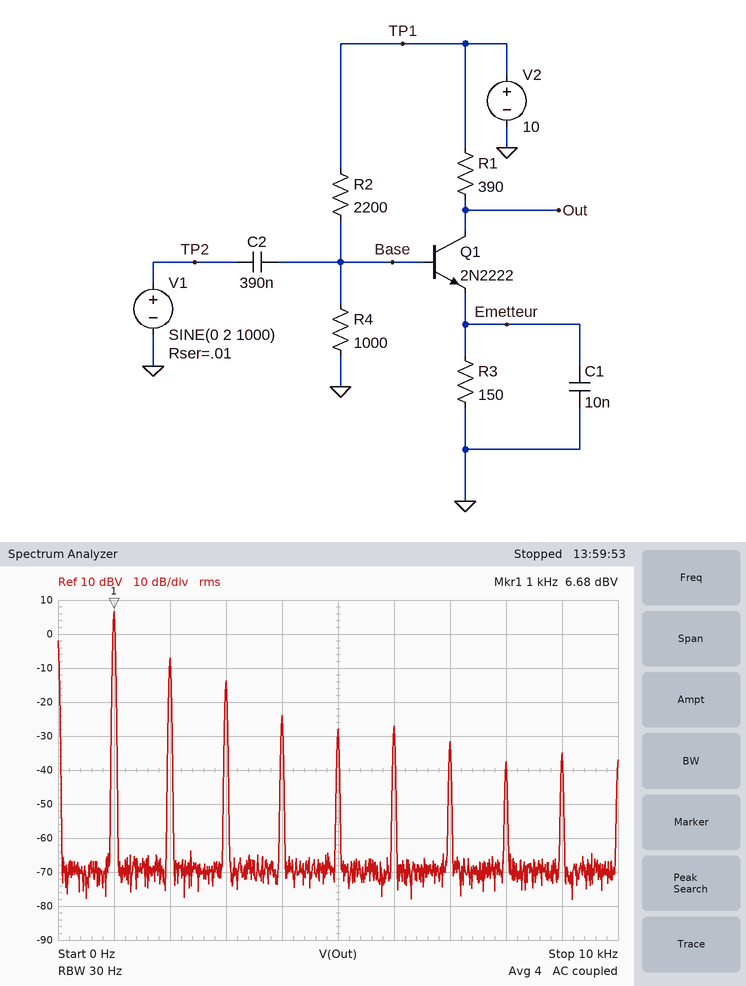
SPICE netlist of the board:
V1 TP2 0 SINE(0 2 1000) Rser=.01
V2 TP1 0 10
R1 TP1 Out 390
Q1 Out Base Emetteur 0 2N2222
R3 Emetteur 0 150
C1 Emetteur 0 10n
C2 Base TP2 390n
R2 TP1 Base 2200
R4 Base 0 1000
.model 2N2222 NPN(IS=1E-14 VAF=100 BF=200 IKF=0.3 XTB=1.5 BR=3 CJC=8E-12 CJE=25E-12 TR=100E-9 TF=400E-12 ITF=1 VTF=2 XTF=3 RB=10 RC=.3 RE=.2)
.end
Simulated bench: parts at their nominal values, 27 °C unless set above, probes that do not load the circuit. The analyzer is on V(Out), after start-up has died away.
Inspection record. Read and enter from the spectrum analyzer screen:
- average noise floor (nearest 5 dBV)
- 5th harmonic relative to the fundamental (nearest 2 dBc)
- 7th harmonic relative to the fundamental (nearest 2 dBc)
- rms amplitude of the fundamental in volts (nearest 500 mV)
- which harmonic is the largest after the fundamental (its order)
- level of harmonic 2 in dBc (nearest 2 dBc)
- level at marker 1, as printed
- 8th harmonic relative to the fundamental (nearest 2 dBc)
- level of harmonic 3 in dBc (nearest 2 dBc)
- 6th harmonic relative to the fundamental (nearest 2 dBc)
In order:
-70 dBV
-34 dBc
-38 dBc
2.0 V
2
-14 dBc
6.68 dBV
-44 dBc
-20 dBc
-34 dBc
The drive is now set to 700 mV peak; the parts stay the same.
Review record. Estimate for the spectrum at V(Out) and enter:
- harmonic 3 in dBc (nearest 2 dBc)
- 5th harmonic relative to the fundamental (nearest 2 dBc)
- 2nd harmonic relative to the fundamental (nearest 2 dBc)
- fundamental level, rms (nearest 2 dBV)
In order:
-28 dBc
-36 dBc
-24 dBc
0 dBV
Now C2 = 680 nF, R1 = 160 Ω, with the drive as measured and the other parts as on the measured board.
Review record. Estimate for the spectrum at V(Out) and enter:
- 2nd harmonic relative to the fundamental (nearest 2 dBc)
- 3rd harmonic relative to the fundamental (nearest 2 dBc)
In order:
-50 dBc
-60 dBc
